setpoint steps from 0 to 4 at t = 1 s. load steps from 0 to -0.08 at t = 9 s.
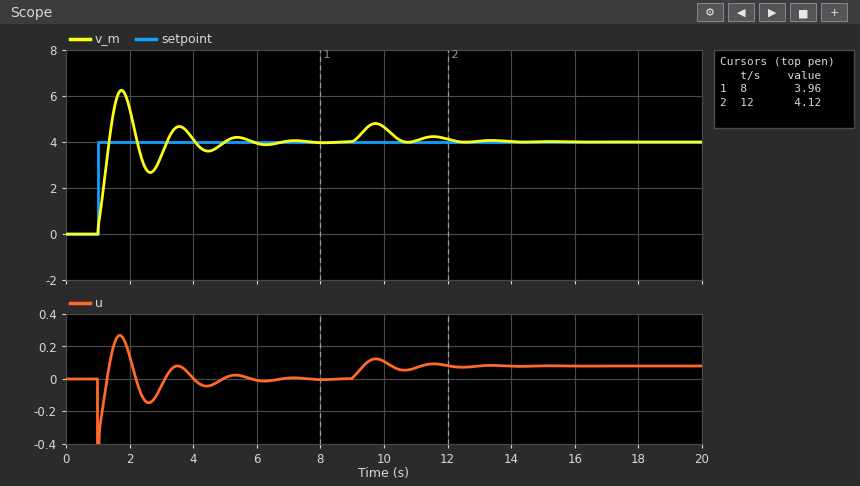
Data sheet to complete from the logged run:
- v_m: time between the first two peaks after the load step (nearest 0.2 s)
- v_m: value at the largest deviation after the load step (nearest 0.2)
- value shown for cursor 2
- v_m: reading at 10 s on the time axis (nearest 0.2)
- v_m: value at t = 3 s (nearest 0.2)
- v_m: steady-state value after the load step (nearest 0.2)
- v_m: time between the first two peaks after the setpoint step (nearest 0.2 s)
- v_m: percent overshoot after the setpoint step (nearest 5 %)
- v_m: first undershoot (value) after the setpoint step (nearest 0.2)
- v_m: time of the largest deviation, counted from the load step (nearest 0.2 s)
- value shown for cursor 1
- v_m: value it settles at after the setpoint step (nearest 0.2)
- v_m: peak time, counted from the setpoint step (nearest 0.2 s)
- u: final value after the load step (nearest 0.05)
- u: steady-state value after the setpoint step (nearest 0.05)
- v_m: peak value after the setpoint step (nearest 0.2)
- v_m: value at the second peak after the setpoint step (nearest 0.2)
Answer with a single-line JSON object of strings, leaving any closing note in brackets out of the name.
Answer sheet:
{"v_m: time between the first two peaks after the load step": "1.8 s", "v_m: value at the largest deviation after the load step": "4.8", "value shown for cursor 2": "4.12", "v_m: reading at 10 s on the time axis": "4.6", "v_m: value at t = 3 s": "3.4", "v_m: steady-state value after the load step": "4.0", "v_m: time between the first two peaks after the setpoint step": "1.8 s", "v_m: percent overshoot after the setpoint step": "55 %", "v_m: first undershoot (value) after the setpoint step": "2.6", "v_m: time of the largest deviation, counted from the load step": "0.8 s", "value shown for cursor 1": "3.96", "v_m: value it settles at after the setpoint step": "4.0", "v_m: peak time, counted from the setpoint step": "0.8 s", "u: final value after the load step": "0.10", "u: steady-state value after the setpoint step": "0.00", "v_m: peak value after the setpoint step": "6.2", "v_m: value at the second peak after the setpoint step": "4.6"}
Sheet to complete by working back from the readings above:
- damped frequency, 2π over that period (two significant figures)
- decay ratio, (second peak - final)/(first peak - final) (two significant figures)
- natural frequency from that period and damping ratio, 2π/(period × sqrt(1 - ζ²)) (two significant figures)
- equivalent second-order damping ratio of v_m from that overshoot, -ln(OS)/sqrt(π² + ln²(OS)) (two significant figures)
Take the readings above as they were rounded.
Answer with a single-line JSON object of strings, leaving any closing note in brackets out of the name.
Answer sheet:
{"damped frequency, 2π over that period": "3.5 rad/s", "decay ratio, (second peak - final)/(first peak - final)": "0.27", "natural frequency from that period and damping ratio, 2π/(period × sqrt(1 - ζ²))": "3.6 rad/s", "equivalent second-order damping ratio of v_m from that overshoot, -ln(OS)/sqrt(π² + ln²(OS))": "0.19"}
